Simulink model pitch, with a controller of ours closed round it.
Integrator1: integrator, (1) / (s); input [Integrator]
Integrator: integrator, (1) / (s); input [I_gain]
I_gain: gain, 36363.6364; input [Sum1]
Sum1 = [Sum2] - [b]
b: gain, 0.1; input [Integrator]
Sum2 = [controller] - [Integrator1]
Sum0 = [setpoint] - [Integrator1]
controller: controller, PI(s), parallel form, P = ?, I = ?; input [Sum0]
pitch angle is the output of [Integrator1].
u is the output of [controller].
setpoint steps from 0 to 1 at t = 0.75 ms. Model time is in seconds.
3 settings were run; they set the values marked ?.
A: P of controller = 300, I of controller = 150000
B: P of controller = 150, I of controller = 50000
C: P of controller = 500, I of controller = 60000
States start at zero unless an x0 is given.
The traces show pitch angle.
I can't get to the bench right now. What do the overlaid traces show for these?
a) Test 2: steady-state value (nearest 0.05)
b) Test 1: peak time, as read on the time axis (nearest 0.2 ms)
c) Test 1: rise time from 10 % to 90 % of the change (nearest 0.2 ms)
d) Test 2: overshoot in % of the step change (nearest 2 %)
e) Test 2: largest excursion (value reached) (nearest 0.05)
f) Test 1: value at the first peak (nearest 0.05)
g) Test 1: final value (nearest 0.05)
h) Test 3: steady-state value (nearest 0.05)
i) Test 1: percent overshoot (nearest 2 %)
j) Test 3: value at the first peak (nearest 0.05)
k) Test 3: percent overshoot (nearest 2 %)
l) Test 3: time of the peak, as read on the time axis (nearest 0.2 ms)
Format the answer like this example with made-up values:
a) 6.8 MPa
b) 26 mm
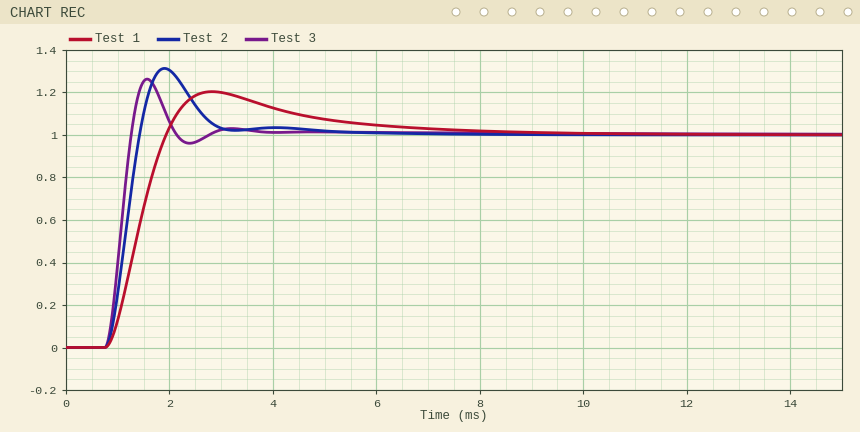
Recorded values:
a) 1.00
b) 2.8 ms
c) 0.8 ms
d) 32 %
e) 1.30
f) 1.20
g) 1.00
h) 1.00
i) 20 %
j) 1.25
k) 26 %
l) 1.6 ms
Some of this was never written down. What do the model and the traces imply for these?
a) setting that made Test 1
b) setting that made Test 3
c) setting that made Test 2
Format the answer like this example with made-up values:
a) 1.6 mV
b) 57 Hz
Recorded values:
a) B
b) C
c) A
